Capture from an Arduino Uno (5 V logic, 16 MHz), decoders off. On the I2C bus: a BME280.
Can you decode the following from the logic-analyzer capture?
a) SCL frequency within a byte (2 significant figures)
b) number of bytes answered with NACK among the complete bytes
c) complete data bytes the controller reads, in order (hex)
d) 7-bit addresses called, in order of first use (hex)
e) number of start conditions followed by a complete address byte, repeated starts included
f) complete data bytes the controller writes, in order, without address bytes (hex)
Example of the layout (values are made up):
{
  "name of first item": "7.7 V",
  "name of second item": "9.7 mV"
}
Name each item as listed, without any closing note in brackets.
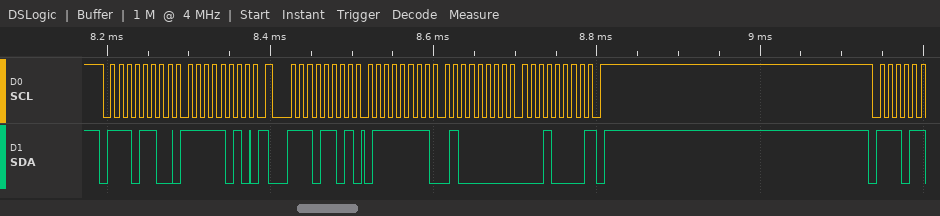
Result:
{
  "SCL frequency within a byte": "100 kHz",
  "number of bytes answered with NACK among the complete bytes": "1",
  "complete data bytes the controller reads, in order": "7F 40 10",
  "7-bit addresses called, in order of first use": "0x76",
  "number of start conditions followed by a complete address byte, repeated starts included": "2",
  "complete data bytes the controller writes, in order, without address bytes": "FA"
}
